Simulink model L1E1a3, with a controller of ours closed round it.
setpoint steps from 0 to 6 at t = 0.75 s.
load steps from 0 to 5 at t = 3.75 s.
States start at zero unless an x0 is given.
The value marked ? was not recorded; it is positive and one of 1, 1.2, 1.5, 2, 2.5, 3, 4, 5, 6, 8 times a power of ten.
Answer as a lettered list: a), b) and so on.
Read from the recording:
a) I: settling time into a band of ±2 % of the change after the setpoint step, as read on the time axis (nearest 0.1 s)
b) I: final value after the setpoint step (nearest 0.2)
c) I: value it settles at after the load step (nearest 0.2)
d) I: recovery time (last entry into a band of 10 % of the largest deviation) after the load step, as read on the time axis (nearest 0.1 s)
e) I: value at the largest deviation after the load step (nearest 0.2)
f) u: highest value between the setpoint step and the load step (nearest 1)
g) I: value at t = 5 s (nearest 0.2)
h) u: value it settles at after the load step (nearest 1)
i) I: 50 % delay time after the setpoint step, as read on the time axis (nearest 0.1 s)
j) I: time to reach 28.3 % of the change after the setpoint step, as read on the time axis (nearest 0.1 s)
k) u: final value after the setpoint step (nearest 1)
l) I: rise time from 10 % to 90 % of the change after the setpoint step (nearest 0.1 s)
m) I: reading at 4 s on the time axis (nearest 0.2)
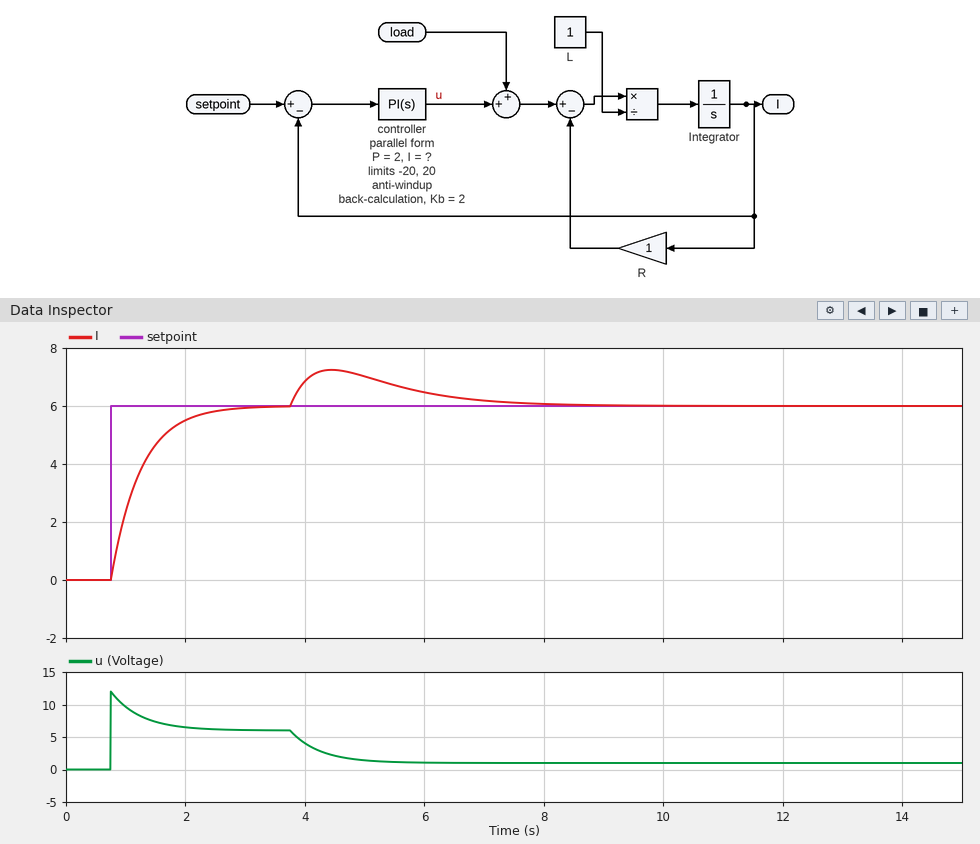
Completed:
a) 2.7 s
b) 6.0
c) 6.0
d) 7.4 s
e) 7.2
f) 12
g) 7.0
h) 1
i) 1.1 s
j) 0.9 s
k) 6
l) 1.1 s
m) 6.8
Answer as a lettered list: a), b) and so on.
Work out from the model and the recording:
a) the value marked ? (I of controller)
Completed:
a) 2
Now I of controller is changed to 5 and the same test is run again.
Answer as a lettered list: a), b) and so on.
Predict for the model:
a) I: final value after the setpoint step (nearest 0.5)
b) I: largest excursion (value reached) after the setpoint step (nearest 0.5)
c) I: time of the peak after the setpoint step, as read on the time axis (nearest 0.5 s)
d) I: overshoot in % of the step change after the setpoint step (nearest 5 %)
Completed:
a) 6.0
b) 6.5
c) 2.0 s
d) 10 %
